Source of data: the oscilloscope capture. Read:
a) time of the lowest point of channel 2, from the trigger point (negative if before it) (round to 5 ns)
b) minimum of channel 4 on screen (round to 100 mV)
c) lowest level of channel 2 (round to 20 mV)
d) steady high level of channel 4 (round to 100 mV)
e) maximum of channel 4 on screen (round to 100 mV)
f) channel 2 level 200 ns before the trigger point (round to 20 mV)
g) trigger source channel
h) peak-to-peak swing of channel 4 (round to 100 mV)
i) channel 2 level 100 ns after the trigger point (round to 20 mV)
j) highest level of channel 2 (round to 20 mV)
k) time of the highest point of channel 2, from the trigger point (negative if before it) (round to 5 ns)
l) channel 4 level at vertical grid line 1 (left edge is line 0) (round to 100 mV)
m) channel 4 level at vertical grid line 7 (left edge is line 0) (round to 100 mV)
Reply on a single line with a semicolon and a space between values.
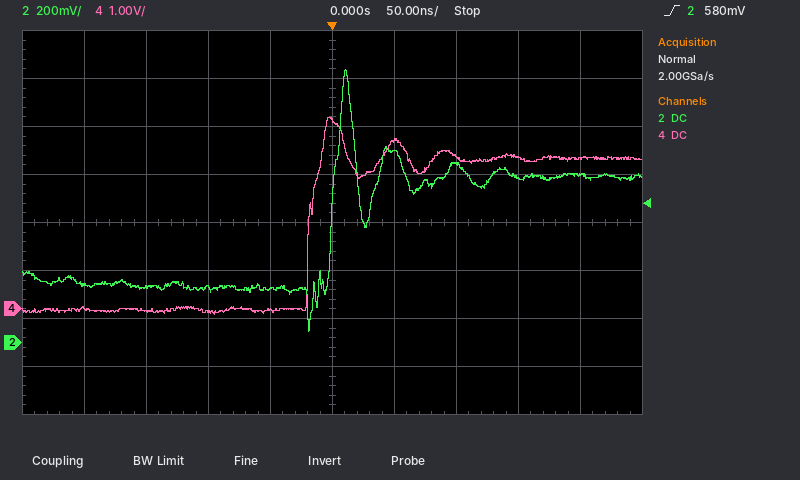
-20 ns; -100 mV; 40 mV; 3.1 V; 4.0 V; 240 mV; channel 2; 4.1 V; 740 mV; 1.14 V; +10 ns; 0.0 V; 3.2 V
